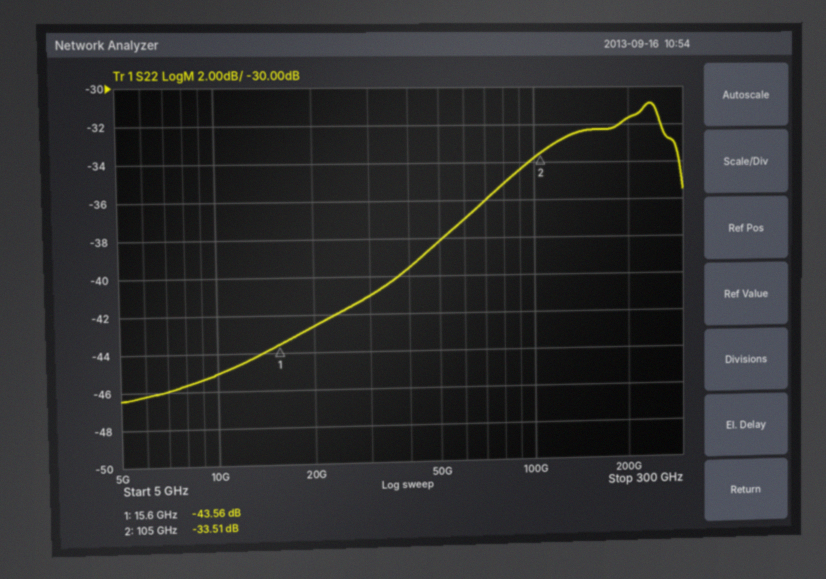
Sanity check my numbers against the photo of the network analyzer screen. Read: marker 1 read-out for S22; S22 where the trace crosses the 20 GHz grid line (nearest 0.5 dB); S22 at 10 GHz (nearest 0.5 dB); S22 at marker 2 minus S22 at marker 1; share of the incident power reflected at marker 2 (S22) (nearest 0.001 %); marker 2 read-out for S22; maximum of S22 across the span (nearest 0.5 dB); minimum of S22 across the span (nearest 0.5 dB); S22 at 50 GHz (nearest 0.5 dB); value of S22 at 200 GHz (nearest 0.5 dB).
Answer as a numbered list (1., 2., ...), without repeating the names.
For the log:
1. -43.56 dB
2. -42.5 dB
3. -45.0 dB
4. 10.05 dB
5. 0.045 %
6. -33.51 dB
7. -31.0 dB
8. -46.5 dB
9. -38.0 dB
10. -31.5 dB
